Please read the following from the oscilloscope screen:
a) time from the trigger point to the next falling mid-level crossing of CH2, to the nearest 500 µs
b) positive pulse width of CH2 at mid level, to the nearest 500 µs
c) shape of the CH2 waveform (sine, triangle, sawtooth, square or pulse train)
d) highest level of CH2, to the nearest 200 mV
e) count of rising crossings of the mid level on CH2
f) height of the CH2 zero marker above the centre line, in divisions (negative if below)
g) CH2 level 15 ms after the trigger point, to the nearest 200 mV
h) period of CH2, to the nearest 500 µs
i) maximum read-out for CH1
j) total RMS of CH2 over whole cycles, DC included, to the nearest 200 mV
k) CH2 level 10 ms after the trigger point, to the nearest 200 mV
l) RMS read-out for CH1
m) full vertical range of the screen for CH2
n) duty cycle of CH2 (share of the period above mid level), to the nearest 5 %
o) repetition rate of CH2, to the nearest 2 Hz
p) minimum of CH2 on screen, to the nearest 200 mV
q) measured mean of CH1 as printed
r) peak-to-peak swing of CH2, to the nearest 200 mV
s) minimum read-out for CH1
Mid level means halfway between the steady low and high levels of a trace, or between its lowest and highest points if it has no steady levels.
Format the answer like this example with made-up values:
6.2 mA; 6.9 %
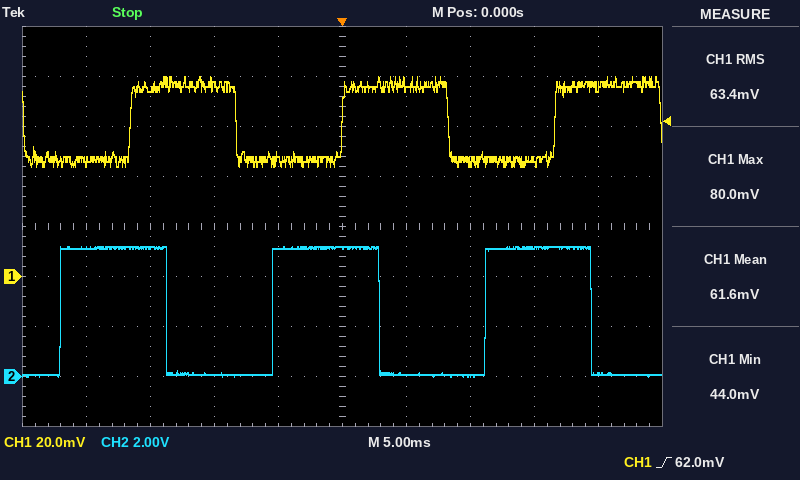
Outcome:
3.0 ms; 8.5 ms; square; 5.2 V; 3; -3.0 div; 5.2 V; 16.5 ms; 80.0 mV; 3.6 V; 0.0 V; 63.4 mV; 16 V; 50 %; 60 Hz; 0.0 V; 61.6 mV; 5.2 V; 44.0 mV
